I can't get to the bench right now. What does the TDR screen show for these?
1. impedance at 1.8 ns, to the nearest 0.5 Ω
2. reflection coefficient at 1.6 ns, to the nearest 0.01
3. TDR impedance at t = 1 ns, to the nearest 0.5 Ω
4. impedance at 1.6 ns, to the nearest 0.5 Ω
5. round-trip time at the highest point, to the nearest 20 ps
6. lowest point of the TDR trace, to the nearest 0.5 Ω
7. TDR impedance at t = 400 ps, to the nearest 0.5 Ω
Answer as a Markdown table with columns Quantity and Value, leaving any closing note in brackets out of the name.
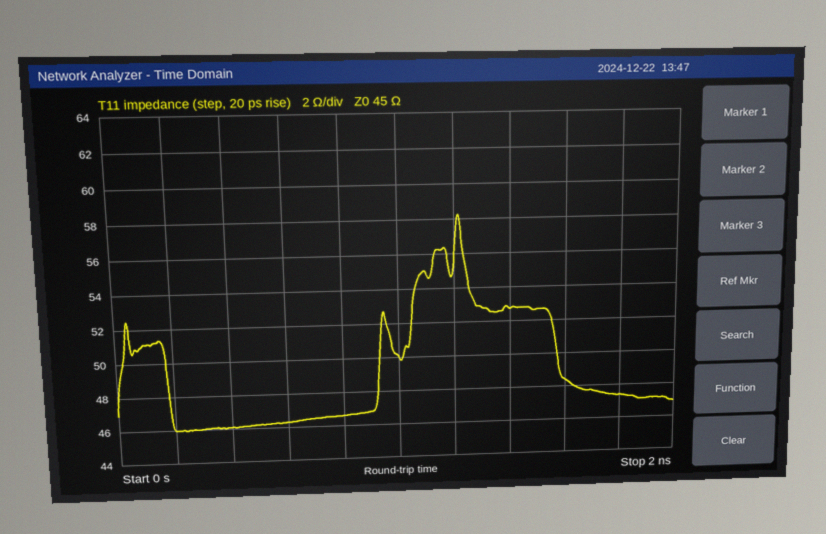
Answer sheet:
| Quantity | Value |
|---|---|
| impedance at 1.8 ns, to the nearest 0.5 Ω | 47.5 Ω |
| reflection coefficient at 1.6 ns, to the nearest 0.01 | +0.04 |
| TDR impedance at t = 1 ns, to the nearest 0.5 Ω | 50.0 Ω |
| impedance at 1.6 ns, to the nearest 0.5 Ω | 48.5 Ω |
| round-trip time at the highest point, to the nearest 20 ps | 1.22 ns |
| lowest point of the TDR trace, to the nearest 0.5 Ω | 46.0 Ω |
| TDR impedance at t = 400 ps, to the nearest 0.5 Ω | 46.0 Ω |
